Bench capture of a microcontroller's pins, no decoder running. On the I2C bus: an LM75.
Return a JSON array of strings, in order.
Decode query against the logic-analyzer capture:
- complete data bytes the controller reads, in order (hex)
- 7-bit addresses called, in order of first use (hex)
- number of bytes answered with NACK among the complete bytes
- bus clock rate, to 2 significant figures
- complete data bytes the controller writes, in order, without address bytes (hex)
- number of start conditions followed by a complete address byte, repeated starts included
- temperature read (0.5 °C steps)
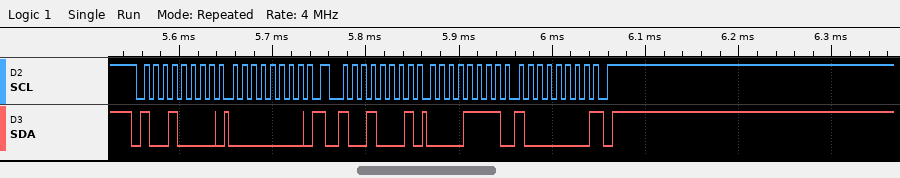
["0F 80", "0x48", "1", "100 kHz", "00", "2", "15.5 °C"]
